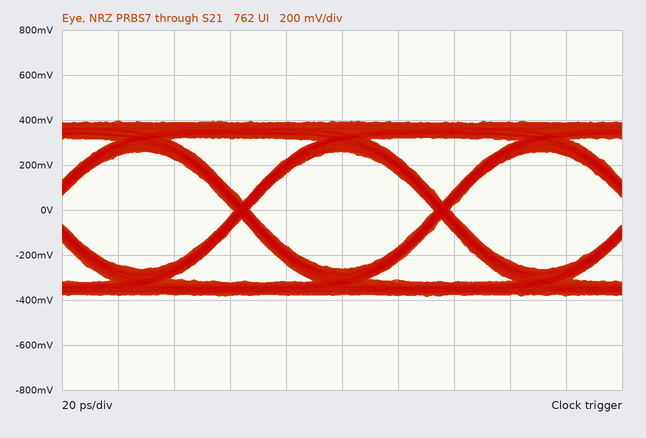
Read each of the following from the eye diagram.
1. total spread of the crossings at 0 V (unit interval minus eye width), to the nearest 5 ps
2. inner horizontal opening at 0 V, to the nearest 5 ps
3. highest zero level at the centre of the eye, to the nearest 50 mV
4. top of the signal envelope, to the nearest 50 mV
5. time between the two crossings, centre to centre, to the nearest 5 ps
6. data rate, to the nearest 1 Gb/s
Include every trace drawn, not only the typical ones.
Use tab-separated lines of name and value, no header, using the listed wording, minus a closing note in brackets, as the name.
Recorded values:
total spread of the crossings at 0 V (unit interval minus eye width), to the nearest 5 ps	5 ps
inner horizontal opening at 0 V, to the nearest 5 ps	65 ps
highest zero level at the centre of the eye, to the nearest 50 mV	-250 mV
top of the signal envelope, to the nearest 50 mV	400 mV
time between the two crossings, centre to centre, to the nearest 5 ps	70 ps
data rate, to the nearest 1 Gb/s	14 Gb/s
